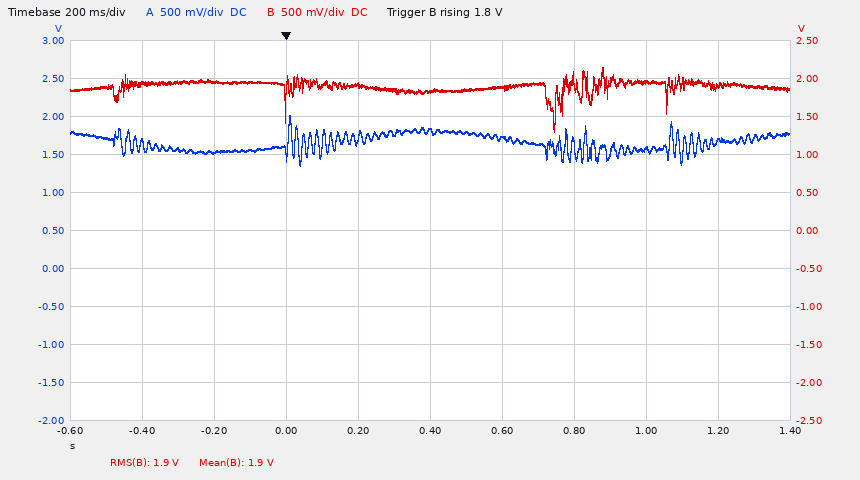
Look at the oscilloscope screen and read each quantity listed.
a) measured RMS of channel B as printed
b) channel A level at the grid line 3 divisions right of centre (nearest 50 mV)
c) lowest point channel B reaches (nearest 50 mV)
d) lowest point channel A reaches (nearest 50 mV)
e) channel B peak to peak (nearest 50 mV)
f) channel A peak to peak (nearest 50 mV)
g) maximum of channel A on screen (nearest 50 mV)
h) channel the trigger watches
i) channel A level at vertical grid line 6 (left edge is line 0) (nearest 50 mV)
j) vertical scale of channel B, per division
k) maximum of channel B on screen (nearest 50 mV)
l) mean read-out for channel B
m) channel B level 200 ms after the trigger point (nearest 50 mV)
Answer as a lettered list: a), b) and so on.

a) 1.9 V
b) 1.55 V
c) 1.30 V
d) 1.35 V
e) 850 mV
f) 650 mV
g) 2.00 V
h) channel B
i) 1.70 V
j) 500 mV
k) 2.15 V
l) 1.9 V
m) 1.90 V
